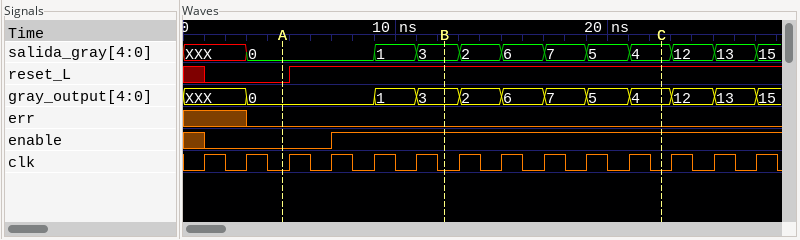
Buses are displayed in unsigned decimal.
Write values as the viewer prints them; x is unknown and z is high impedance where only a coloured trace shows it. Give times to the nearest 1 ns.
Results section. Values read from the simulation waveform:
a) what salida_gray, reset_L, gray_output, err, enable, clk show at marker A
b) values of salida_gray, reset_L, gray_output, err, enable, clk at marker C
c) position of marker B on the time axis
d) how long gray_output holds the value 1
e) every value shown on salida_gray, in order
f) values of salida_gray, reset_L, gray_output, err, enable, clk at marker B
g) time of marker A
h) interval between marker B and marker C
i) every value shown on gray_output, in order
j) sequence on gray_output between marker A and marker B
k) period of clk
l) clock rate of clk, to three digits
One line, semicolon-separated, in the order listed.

salida_gray=0, reset_L=0, gray_output=0, err=0, enable=0, clk=0; salida_gray=4, reset_L=1, gray_output=4, err=0, enable=1, clk=0; 12 ns; 2 ns; XXX, 0, 1, 3, 2, 6, 7, 5, 4, 12, 13, 15; salida_gray=3, reset_L=1, gray_output=3, err=0, enable=1, clk=0; 5 ns; 10 ns; XXX, 0, 1, 3, 2, 6, 7, 5, 4, 12, 13, 15; 0, 1, 3; 2 ns; 500 MHz
